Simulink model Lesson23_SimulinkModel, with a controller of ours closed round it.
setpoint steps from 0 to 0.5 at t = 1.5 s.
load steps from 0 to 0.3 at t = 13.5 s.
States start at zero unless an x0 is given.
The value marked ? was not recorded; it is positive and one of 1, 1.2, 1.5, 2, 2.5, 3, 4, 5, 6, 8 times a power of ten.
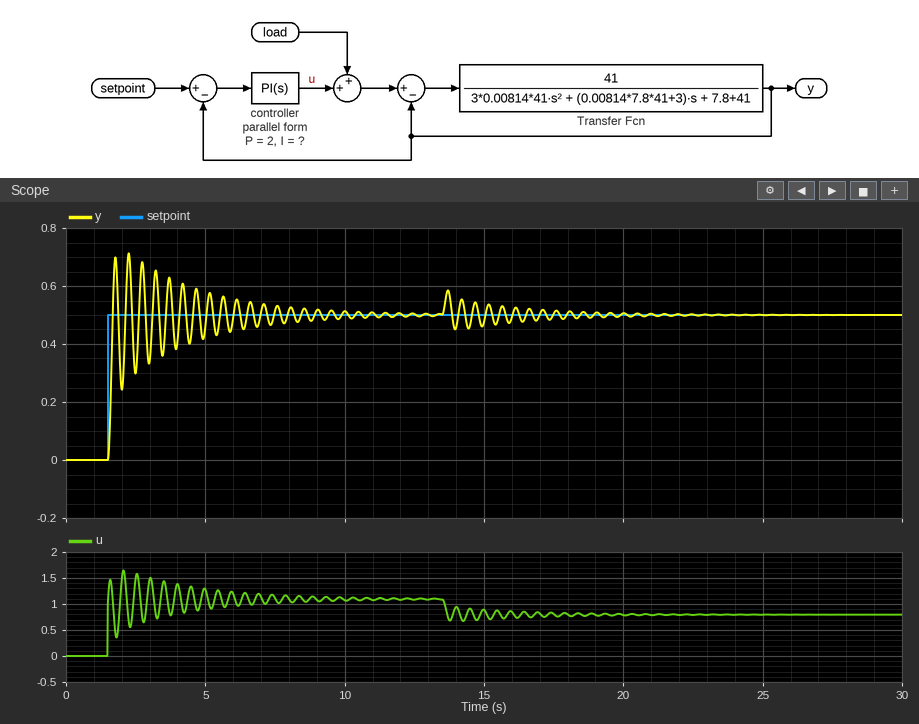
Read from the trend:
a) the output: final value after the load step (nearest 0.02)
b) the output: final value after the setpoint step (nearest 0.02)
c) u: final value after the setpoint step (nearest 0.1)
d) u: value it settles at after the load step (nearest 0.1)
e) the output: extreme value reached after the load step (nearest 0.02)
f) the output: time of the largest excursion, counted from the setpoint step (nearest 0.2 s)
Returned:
0.50
0.50
1.1
0.8
0.58
0.8 s
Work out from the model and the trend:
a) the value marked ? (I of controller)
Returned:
20
